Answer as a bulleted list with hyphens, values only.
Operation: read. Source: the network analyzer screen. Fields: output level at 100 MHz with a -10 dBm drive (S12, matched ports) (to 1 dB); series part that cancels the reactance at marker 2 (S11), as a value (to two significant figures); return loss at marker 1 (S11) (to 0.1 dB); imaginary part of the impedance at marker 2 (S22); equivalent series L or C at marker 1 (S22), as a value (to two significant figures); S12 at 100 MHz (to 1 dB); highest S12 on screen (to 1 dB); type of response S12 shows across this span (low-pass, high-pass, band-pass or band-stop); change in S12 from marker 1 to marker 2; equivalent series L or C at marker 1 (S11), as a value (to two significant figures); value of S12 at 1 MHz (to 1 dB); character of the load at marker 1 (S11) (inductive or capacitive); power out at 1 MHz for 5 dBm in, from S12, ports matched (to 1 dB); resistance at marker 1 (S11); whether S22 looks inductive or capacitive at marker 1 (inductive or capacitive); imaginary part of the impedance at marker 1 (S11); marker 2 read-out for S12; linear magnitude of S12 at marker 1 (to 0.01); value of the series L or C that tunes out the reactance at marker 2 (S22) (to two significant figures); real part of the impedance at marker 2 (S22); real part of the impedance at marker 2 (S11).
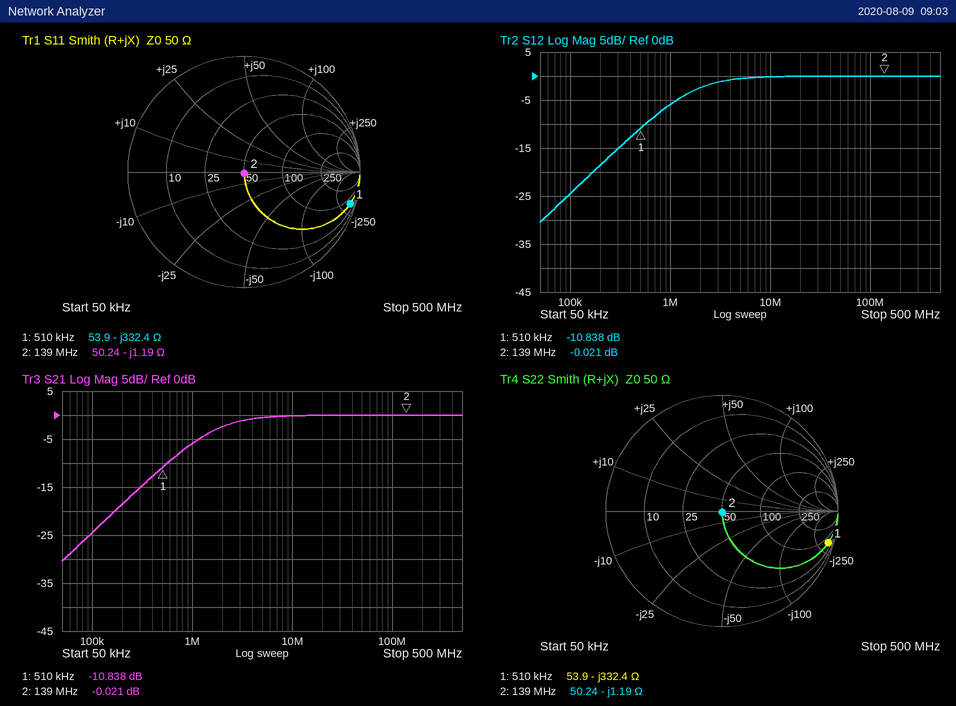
- -10 dBm
- 1.4 nH
- 0.4 dB
- -1.19 Ω
- 940 pF
- 0 dB
- 0 dB
- high-pass
- 10.817 dB
- 940 pF
- -6 dB
- capacitive
- -1 dBm
- 53.9 Ω
- capacitive
- -332.4 Ω
- -0.021 dB
- 0.29
- 1.4 nH
- 50.24 Ω
- 50.24 Ω
